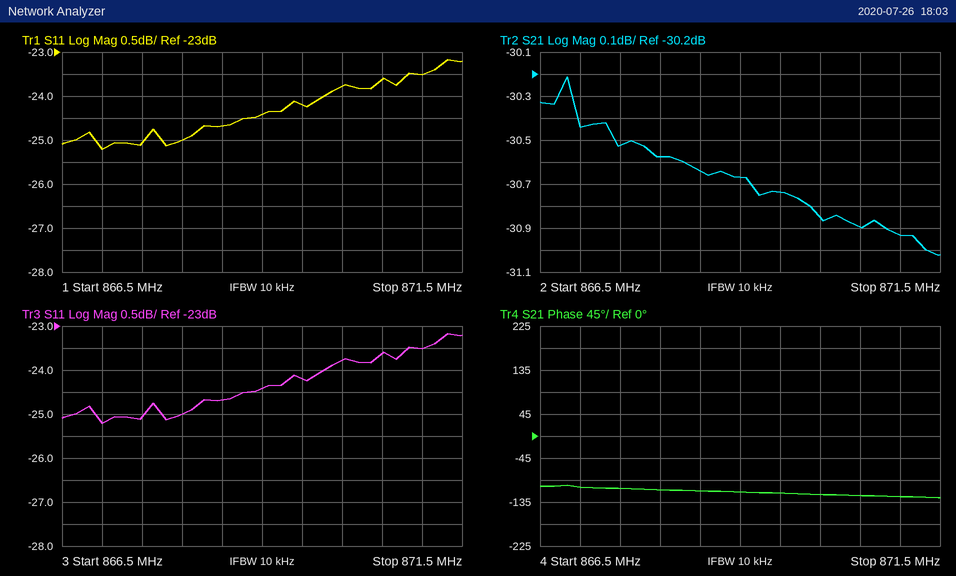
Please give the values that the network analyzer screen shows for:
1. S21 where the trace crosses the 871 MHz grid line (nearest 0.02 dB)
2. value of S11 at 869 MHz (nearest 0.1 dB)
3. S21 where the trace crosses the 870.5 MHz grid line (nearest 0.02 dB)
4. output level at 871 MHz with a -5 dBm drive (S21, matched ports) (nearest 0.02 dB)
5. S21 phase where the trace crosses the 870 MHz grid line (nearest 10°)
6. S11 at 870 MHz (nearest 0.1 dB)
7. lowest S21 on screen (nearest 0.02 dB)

-30.94 dB
-24.4 dB
-30.90 dB
-35.94 dBm
-120°
-23.8 dB
-31.02 dB
